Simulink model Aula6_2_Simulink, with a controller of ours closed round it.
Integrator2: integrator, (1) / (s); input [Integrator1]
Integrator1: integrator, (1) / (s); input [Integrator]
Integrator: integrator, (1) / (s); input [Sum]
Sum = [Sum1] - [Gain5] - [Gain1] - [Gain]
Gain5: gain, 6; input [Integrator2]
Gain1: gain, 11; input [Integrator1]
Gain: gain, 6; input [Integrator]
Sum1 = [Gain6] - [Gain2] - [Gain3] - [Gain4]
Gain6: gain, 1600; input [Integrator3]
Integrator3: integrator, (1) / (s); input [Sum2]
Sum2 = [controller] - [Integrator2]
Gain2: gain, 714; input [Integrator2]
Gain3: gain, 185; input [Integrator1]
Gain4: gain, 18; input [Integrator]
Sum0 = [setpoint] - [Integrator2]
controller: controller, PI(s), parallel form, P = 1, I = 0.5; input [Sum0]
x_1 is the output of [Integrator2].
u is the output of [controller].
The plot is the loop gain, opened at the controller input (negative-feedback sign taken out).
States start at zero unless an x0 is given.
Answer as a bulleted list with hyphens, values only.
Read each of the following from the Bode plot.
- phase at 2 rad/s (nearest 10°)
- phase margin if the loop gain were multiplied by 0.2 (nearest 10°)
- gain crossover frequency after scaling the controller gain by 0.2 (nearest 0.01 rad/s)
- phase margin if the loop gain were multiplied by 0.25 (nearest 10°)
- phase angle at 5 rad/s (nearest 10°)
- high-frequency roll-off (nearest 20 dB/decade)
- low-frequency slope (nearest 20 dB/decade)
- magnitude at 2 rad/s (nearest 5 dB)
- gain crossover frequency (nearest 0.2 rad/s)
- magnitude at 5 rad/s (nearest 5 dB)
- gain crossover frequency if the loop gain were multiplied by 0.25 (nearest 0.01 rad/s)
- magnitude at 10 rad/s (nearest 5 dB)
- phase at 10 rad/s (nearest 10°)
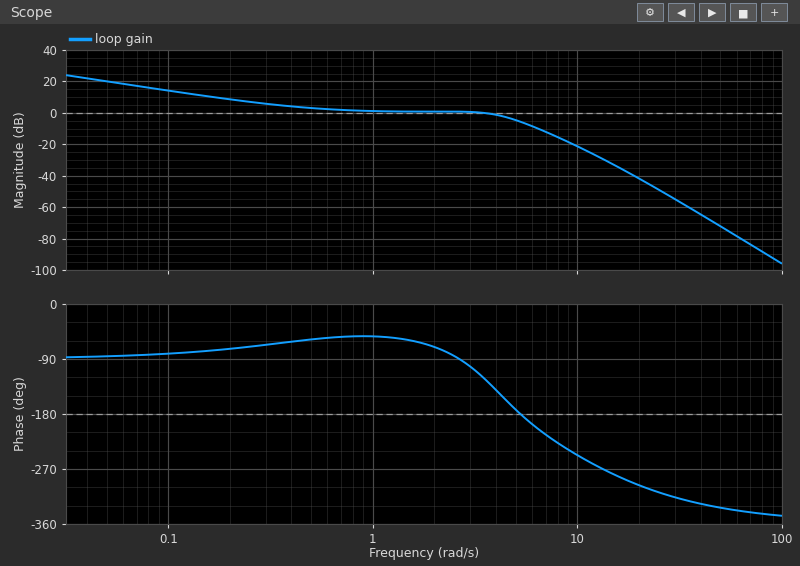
- -70°
- 100°
- 0.10 rad/s
- 100°
- -170°
- -80 dB/decade
- -20 dB/decade
- 0 dB
- 3.4 rad/s
- -5 dB
- 0.13 rad/s
- -20 dB
- -250°
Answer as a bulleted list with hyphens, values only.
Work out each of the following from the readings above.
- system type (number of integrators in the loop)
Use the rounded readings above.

- 1
